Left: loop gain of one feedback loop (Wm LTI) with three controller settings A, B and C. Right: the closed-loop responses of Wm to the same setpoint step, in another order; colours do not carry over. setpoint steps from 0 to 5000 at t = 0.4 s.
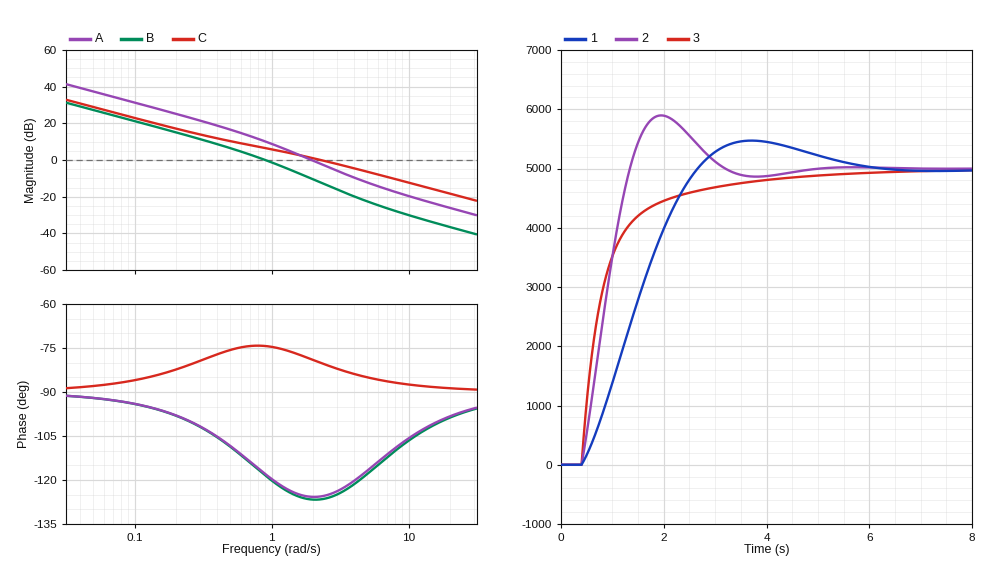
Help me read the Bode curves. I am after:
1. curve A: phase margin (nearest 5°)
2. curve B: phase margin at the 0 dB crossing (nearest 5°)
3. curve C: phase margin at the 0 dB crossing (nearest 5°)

55°
60°
100°
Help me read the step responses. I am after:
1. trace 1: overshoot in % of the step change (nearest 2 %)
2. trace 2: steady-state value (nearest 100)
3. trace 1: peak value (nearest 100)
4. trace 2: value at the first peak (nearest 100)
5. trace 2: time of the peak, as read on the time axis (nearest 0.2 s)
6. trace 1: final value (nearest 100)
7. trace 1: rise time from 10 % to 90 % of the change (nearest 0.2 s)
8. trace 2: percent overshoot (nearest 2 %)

10 %
5000
5500
5900
2.0 s
5000
1.6 s
18 %
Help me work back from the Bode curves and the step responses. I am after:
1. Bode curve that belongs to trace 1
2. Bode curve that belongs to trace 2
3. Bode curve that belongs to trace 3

B
A
C
